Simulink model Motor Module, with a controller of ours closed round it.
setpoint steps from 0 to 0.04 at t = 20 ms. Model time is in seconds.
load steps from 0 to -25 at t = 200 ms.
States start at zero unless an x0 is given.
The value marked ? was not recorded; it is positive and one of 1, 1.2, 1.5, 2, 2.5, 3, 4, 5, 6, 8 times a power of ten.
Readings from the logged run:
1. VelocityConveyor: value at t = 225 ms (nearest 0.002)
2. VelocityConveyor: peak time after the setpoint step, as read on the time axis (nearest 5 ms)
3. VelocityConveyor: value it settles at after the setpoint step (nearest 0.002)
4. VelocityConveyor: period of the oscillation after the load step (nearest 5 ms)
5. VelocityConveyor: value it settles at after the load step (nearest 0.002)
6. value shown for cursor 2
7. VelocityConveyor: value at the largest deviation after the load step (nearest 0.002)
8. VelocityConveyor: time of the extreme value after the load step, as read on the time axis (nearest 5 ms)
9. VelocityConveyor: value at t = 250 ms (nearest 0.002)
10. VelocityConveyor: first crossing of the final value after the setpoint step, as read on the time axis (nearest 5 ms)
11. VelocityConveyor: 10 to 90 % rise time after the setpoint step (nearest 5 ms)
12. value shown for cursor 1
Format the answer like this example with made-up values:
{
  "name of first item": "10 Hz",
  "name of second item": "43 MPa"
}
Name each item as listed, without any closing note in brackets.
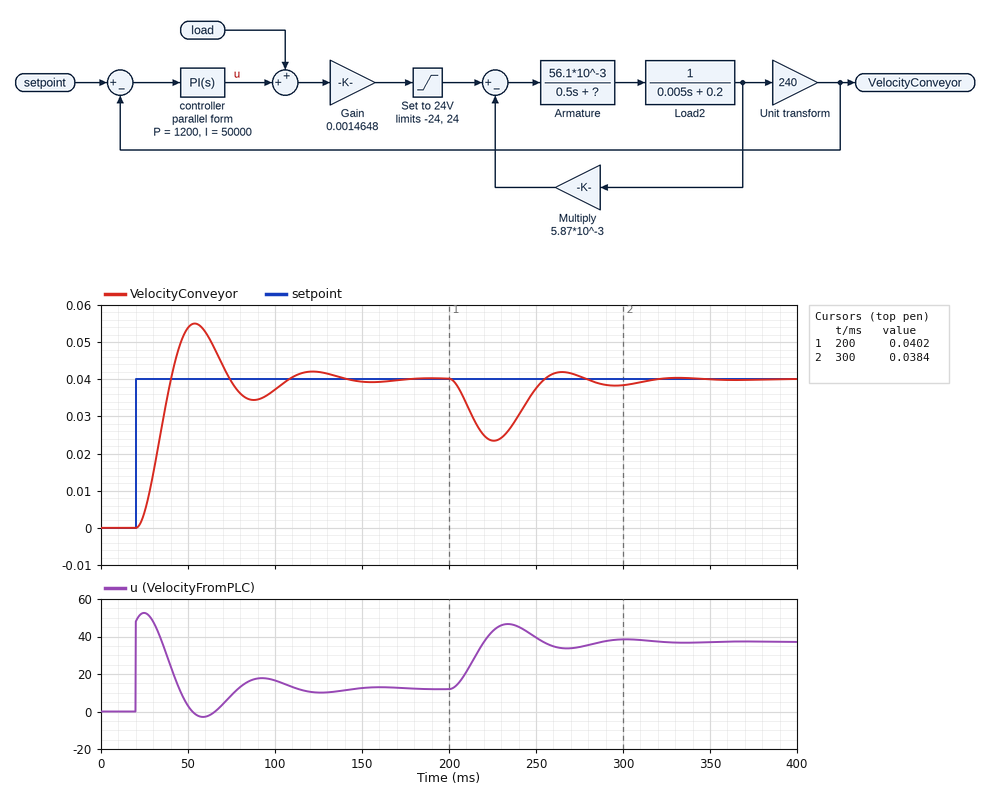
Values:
{
  "VelocityConveyor: value at t = 225 ms": "0.024",
  "VelocityConveyor: peak time after the setpoint step, as read on the time axis": "55 ms",
  "VelocityConveyor: value it settles at after the setpoint step": "0.040",
  "VelocityConveyor: period of the oscillation after the load step": "70 ms",
  "VelocityConveyor: value it settles at after the load step": "0.040",
  "value shown for cursor 2": "0.0384",
  "VelocityConveyor: value at the largest deviation after the load step": "0.024",
  "VelocityConveyor: time of the extreme value after the load step, as read on the time axis": "225 ms",
  "VelocityConveyor: value at t = 250 ms": "0.038",
  "VelocityConveyor: first crossing of the final value after the setpoint step, as read on the time axis": "40 ms",
  "VelocityConveyor: 10 to 90 % rise time after the setpoint step": "15 ms",
  "value shown for cursor 1": "0.0402"
}
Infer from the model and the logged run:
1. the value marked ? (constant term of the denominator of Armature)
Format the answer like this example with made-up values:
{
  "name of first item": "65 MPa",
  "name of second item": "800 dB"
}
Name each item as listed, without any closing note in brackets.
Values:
{
  "the value marked ?": "30"
}
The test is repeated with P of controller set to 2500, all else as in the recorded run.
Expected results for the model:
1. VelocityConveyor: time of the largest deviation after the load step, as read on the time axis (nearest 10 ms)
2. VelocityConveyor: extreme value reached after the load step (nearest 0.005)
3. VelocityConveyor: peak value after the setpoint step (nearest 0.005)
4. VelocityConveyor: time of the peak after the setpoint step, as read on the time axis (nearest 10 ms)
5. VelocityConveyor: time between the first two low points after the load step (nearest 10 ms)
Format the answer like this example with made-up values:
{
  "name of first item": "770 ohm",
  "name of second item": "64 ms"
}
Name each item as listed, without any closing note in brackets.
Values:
{
  "VelocityConveyor: time of the largest deviation after the load step, as read on the time axis": "220 ms",
  "VelocityConveyor: extreme value reached after the load step": "0.030",
  "VelocityConveyor: peak value after the setpoint step": "0.055",
  "VelocityConveyor: time of the peak after the setpoint step, as read on the time axis": "40 ms",
  "VelocityConveyor: time between the first two low points after the load step": "40 ms"
}
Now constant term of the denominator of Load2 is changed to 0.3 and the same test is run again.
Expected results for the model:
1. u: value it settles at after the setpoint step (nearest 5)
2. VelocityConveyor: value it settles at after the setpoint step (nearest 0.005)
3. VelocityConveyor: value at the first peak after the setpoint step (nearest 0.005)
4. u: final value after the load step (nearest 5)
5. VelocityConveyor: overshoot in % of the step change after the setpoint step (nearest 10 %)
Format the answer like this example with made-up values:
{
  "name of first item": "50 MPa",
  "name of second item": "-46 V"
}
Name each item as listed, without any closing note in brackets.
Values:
{
  "u: value it settles at after the setpoint step": "20",
  "VelocityConveyor: value it settles at after the setpoint step": "0.040",
  "VelocityConveyor: value at the first peak after the setpoint step": "0.050",
  "u: final value after the load step": "45",
  "VelocityConveyor: overshoot in % of the step change after the setpoint step": "20 %"
}
